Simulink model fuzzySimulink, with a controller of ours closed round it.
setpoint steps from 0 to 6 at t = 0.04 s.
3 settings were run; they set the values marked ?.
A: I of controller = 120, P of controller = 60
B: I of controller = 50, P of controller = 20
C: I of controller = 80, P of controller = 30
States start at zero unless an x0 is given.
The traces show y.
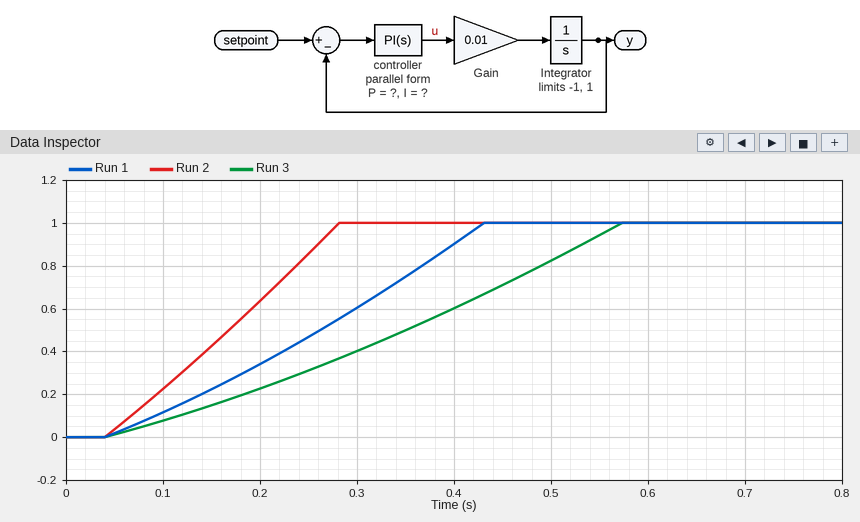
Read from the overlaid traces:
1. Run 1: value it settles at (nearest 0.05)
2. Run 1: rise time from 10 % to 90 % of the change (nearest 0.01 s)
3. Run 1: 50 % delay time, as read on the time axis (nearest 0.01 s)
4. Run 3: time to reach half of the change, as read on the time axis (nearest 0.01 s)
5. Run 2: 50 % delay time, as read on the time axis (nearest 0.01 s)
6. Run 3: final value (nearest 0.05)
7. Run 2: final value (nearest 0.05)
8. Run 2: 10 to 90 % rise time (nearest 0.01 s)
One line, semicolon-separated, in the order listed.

1.00; 0.31 s; 0.26 s; 0.35 s; 0.17 s; 1.00; 1.00; 0.19 s
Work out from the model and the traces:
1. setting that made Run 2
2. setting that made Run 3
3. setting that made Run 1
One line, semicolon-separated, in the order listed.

A; B; C
